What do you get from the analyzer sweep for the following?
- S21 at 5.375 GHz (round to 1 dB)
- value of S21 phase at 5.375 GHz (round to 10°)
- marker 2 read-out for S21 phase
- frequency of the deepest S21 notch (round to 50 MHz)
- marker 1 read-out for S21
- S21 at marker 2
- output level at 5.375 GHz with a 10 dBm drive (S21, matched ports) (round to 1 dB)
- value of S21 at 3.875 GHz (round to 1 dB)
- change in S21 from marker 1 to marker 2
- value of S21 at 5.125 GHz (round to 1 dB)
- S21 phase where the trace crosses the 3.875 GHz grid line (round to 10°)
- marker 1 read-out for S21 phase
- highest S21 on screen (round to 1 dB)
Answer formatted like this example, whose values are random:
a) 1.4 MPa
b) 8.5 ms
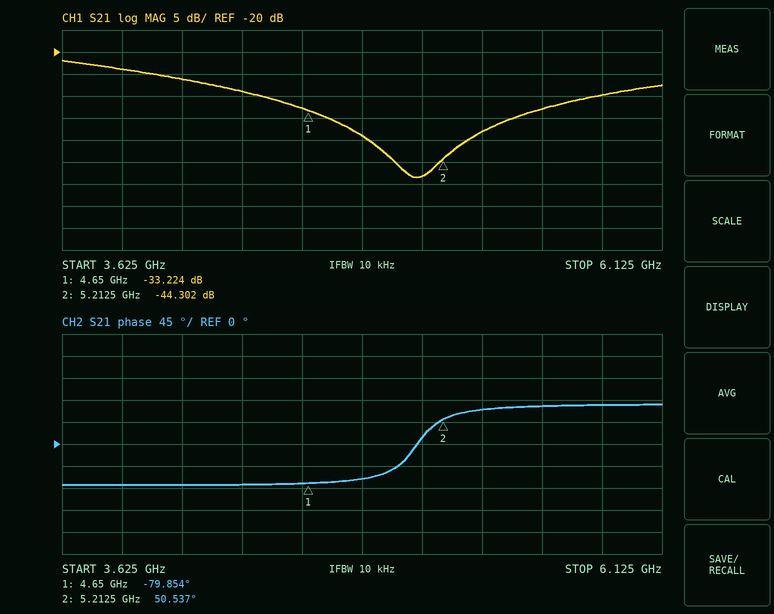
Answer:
a) -38 dB
b) 70°
c) 50.537°
d) 5.10 GHz
e) -33.224 dB
f) -44.302 dB
g) -28 dBm
h) -24 dB
i) -11.078 dB
j) -48 dB
k) -80°
l) -79.854°
m) -22 dB
